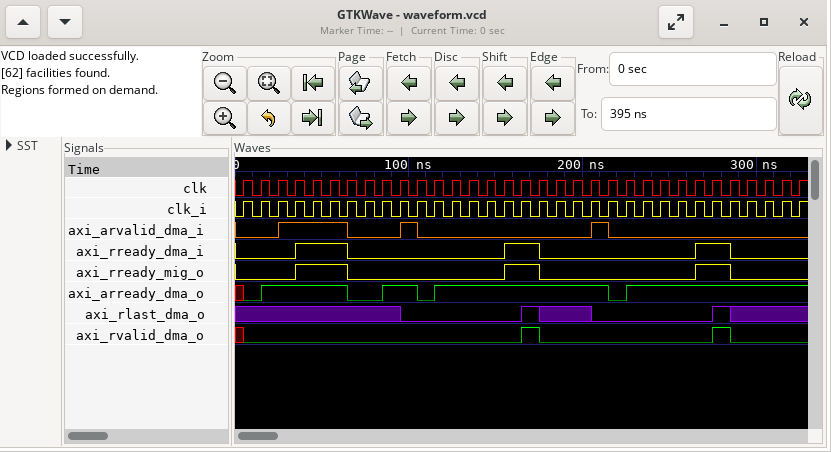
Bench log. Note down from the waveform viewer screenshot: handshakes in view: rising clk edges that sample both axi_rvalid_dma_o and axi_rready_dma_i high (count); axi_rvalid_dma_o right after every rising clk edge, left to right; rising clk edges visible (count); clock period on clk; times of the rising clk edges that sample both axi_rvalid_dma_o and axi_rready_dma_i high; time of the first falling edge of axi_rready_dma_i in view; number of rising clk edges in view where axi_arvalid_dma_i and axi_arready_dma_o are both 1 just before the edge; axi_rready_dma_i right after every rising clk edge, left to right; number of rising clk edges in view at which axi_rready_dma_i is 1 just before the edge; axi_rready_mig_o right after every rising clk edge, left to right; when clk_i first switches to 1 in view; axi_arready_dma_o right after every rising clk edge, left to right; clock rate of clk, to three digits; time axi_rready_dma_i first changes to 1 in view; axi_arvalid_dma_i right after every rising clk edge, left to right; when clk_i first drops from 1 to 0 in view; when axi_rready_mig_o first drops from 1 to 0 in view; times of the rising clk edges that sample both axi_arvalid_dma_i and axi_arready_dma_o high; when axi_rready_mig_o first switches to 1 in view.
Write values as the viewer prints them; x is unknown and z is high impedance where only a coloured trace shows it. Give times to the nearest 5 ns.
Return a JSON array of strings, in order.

["2", "0 0 0 0 0 0 0 0 0 0 0 0 0 0 0 0 1 0 0 0 0 0 0 0 0 0 0 1 0 0 0 0 0", "33", "10 ns", "175 ns, 285 ns", "65 ns", "6", "0 0 0 1 1 1 0 0 0 0 0 0 0 0 0 1 1 0 0 0 0 0 0 0 0 0 1 1 0 0 0 0 0", "7", "0 0 0 1 1 1 0 0 0 0 0 0 0 0 0 1 1 0 0 0 0 0 0 0 0 0 1 1 0 0 0 0 0", "5 ns", "0 1 1 1 1 1 0 0 1 1 0 1 1 1 1 1 1 1 1 1 1 0 1 1 1 1 1 1 1 1 1 1 1", "100 MHz", "35 ns", "0 0 1 1 1 1 0 0 0 1 0 0 0 0 0 0 0 0 0 0 1 0 0 0 0 0 0 0 0 0 0 0 0", "10 ns", "65 ns", "35 ns, 45 ns, 55 ns, 65 ns, 105 ns, 215 ns", "35 ns"]
